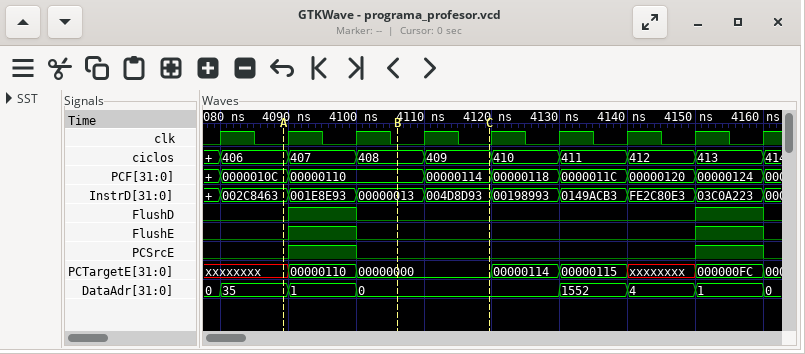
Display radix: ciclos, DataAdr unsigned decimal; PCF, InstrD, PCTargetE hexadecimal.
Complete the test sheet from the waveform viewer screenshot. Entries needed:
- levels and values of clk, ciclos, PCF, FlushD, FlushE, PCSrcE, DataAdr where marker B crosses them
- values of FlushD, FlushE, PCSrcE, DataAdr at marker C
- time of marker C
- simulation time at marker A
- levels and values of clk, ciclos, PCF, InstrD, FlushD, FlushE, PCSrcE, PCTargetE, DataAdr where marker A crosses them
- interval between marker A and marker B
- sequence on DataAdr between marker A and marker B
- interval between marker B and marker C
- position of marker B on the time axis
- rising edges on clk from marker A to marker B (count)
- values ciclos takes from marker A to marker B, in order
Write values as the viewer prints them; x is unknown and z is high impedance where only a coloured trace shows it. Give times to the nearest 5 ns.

clk=0, ciclos=408, PCF=00000110, FlushD=0, FlushE=0, PCSrcE=0, DataAdr=0
FlushD=0, FlushE=0, PCSrcE=0, DataAdr=0
4120 ns
4090 ns
clk=0, ciclos=406, PCF=0000010C, InstrD=002C8463, FlushD=0, FlushE=0, PCSrcE=0, PCTargetE=xxxxxxxx, DataAdr=35
15 ns
35, 1, 0
15 ns
4105 ns
2
406, 407, 408
